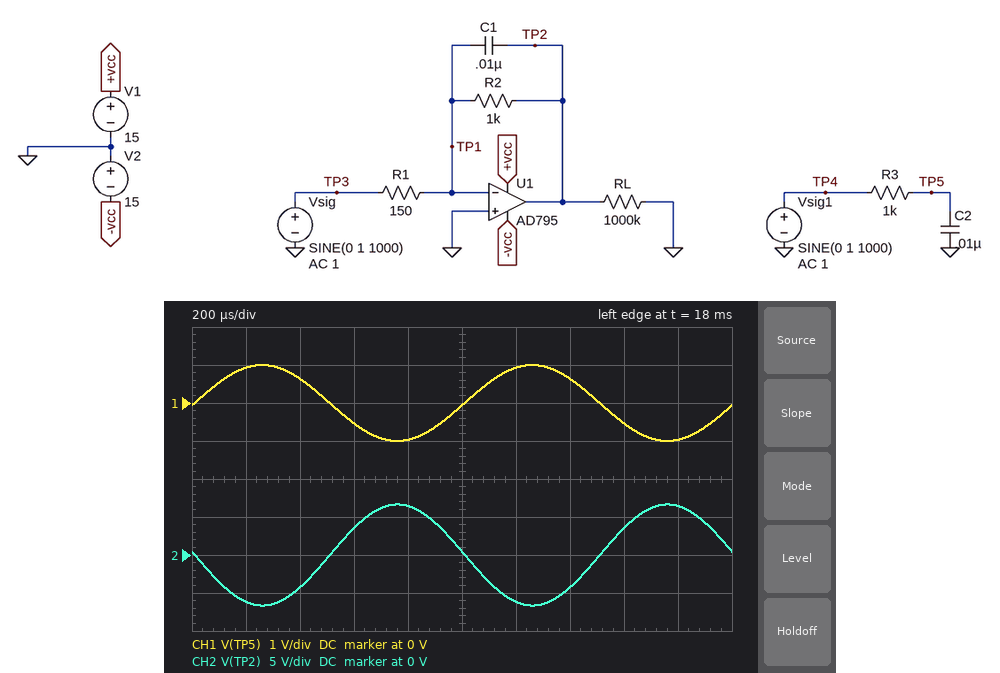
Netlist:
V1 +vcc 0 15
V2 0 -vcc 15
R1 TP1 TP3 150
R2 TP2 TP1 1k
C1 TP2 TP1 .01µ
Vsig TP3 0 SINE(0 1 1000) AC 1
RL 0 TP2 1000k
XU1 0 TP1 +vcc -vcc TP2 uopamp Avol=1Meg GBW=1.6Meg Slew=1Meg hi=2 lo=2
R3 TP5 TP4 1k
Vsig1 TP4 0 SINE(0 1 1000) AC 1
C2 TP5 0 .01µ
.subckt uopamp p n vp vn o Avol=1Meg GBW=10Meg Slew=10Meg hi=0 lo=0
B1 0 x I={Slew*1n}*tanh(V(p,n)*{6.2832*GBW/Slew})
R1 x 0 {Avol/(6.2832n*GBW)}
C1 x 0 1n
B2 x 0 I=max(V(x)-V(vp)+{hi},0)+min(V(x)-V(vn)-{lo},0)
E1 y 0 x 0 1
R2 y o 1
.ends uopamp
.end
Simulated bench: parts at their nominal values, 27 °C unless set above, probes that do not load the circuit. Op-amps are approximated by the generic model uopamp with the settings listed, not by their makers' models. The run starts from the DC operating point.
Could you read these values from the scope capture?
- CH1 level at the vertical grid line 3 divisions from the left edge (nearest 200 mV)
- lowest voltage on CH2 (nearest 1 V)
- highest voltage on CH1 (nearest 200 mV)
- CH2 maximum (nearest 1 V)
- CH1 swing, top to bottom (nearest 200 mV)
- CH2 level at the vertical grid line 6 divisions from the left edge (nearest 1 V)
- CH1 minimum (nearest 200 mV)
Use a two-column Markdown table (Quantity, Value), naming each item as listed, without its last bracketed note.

| Quantity | Value |
|---|---|
| CH1 level at the vertical grid line 3 divisions from the left edge | -600 mV |
| lowest voltage on CH2 | -7 V |
| highest voltage on CH1 | 1.0 V |
| CH2 maximum | 7 V |
| CH1 swing, top to bottom | 2.0 V |
| CH2 level at the vertical grid line 6 divisions from the left edge | -6 V |
| CH1 minimum | -1.0 V |
